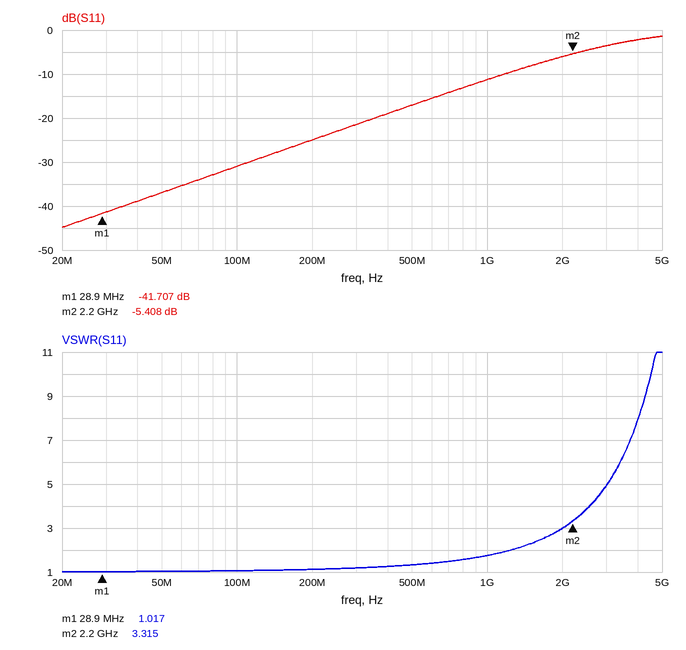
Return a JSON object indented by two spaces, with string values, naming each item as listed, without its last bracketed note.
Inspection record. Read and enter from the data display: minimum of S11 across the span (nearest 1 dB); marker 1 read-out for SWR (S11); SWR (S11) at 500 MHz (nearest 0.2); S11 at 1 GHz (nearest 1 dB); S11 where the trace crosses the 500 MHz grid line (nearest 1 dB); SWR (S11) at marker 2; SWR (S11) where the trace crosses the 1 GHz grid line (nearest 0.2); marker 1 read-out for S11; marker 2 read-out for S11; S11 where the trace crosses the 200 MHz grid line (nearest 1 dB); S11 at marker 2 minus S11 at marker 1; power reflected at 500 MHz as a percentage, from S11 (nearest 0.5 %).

{
  "minimum of S11 across the span": "-45 dB",
  "marker 1 read-out for SWR": "1.017",
  "SWR (S11) at 500 MHz": "1.4",
  "S11 at 1 GHz": "-11 dB",
  "S11 where the trace crosses the 500 MHz grid line": "-17 dB",
  "SWR (S11) at marker 2": "3.315",
  "SWR (S11) where the trace crosses the 1 GHz grid line": "1.8",
  "marker 1 read-out for S11": "-41.707 dB",
  "marker 2 read-out for S11": "-5.408 dB",
  "S11 where the trace crosses the 200 MHz grid line": "-25 dB",
  "S11 at marker 2 minus S11 at marker 1": "36.299 dB",
  "power reflected at 500 MHz as a percentage, from S11": "2.0 %"
}
